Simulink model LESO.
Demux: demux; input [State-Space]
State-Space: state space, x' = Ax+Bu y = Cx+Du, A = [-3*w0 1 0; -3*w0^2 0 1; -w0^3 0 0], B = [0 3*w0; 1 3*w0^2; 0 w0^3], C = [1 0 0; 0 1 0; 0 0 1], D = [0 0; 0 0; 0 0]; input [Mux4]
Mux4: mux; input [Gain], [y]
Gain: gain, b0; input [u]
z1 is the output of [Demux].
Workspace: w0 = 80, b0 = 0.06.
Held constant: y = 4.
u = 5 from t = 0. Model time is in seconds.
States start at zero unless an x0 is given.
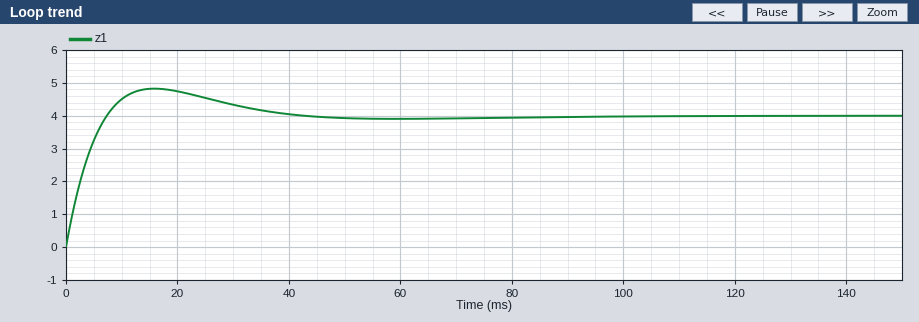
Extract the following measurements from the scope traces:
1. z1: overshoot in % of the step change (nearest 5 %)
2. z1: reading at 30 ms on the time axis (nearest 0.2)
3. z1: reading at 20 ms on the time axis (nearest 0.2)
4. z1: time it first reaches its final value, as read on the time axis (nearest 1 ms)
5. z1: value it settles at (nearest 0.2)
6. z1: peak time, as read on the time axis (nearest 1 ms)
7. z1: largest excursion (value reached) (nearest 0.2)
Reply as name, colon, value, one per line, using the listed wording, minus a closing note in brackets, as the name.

z1: overshoot in % of the step change: 20 %
z1: reading at 30 ms on the time axis: 4.4
z1: reading at 20 ms on the time axis: 4.8
z1: time it first reaches its final value, as read on the time axis: 7 ms
z1: value it settles at: 4.0
z1: peak time, as read on the time axis: 16 ms
z1: largest excursion (value reached): 4.8
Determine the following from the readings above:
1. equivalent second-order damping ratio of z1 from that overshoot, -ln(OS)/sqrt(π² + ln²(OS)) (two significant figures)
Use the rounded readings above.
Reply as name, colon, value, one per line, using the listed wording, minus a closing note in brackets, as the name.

equivalent second-order damping ratio of z1 from that overshoot, -ln(OS)/sqrt(π² + ln²(OS)): 0.46
